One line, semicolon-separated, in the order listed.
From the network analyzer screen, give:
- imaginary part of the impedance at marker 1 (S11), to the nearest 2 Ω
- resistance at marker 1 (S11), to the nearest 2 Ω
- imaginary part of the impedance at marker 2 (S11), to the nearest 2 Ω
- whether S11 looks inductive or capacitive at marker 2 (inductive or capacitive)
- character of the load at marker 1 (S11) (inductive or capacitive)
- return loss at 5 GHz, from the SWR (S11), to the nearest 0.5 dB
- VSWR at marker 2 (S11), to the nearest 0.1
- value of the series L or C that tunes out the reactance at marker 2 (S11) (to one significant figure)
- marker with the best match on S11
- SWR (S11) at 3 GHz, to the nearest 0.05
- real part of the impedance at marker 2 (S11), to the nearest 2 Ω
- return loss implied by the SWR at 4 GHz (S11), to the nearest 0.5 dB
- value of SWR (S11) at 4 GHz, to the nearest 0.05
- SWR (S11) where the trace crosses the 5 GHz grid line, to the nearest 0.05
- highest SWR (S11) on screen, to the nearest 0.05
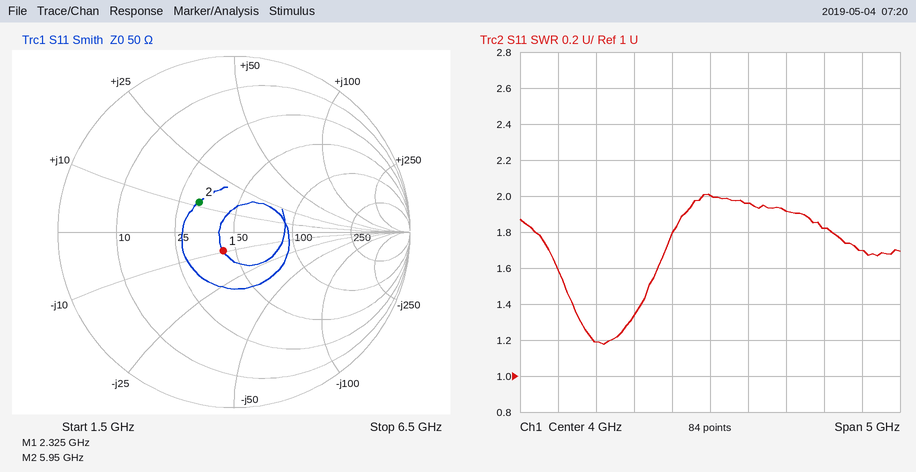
-10 Ω; 44 Ω; +12 Ω; inductive; capacitive; 10.0 dB; 1.7; 2 pF; marker 1; 1.35; 32 Ω; 9.5 dB; 2.00; 1.90; 2.00
